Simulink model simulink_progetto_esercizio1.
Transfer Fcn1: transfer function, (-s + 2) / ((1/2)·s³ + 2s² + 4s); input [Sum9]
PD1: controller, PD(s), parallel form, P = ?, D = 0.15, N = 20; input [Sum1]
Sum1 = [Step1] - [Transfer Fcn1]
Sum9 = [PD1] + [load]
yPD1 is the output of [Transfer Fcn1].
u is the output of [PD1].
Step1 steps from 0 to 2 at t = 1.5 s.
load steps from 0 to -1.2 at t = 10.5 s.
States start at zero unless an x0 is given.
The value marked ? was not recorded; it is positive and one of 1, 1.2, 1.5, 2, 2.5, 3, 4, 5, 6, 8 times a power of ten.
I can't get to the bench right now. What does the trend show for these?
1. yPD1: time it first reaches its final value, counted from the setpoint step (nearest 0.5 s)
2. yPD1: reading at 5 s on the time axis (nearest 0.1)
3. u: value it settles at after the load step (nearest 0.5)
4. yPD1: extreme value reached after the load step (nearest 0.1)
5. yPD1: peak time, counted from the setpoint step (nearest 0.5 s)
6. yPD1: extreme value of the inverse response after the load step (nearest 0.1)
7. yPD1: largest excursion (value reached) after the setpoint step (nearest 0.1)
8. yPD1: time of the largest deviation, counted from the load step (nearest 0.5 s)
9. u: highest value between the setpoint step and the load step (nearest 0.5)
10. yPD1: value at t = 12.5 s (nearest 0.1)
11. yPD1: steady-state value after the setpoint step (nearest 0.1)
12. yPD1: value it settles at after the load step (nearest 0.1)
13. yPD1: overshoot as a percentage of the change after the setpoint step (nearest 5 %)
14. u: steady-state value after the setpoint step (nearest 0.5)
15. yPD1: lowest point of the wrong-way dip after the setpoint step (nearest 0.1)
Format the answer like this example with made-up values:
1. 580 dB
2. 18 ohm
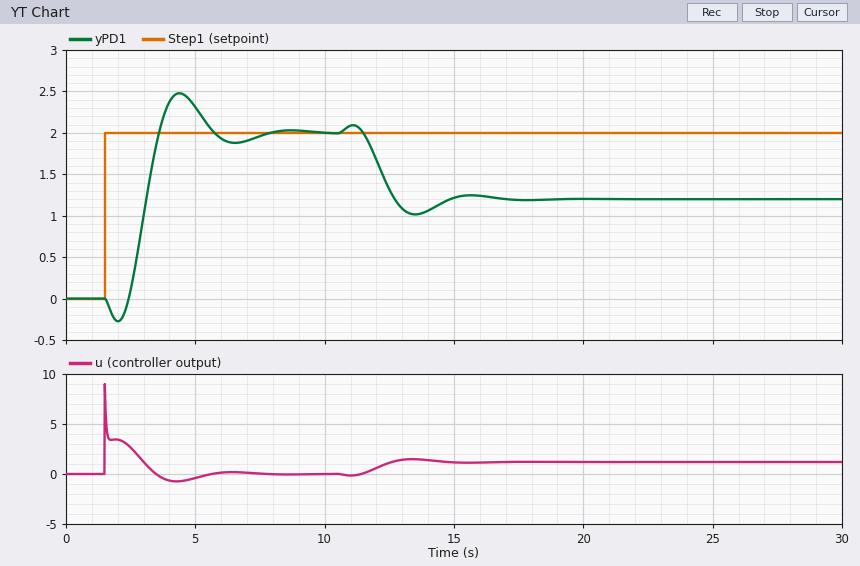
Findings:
1. 2.0 s
2. 2.3
3. 1.0
4. 1.0
5. 3.0 s
6. 2.1
7. 2.5
8. 3.0 s
9. 9.0
10. 1.3
11. 2.0
12. 1.2
13. 25 %
14. 0.0
15. -0.3
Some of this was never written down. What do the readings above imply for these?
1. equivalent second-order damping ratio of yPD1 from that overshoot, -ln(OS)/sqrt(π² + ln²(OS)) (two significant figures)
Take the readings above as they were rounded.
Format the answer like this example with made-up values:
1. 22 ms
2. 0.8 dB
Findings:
1. 0.40
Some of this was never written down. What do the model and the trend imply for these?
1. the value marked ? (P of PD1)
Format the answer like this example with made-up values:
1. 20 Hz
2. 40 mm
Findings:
1. 1.5
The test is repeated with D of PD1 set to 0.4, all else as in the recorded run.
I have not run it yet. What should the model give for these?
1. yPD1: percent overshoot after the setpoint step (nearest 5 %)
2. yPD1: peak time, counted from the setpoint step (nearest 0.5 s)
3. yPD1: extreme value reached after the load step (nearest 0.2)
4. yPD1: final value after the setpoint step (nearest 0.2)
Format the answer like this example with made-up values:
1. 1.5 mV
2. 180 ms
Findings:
1. 15 %
2. 2.5 s
3. 1.2
4. 2.0
